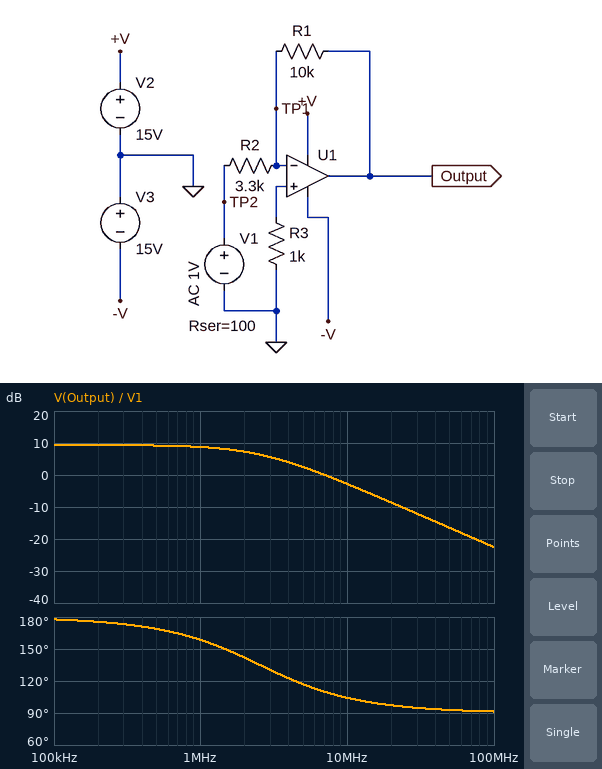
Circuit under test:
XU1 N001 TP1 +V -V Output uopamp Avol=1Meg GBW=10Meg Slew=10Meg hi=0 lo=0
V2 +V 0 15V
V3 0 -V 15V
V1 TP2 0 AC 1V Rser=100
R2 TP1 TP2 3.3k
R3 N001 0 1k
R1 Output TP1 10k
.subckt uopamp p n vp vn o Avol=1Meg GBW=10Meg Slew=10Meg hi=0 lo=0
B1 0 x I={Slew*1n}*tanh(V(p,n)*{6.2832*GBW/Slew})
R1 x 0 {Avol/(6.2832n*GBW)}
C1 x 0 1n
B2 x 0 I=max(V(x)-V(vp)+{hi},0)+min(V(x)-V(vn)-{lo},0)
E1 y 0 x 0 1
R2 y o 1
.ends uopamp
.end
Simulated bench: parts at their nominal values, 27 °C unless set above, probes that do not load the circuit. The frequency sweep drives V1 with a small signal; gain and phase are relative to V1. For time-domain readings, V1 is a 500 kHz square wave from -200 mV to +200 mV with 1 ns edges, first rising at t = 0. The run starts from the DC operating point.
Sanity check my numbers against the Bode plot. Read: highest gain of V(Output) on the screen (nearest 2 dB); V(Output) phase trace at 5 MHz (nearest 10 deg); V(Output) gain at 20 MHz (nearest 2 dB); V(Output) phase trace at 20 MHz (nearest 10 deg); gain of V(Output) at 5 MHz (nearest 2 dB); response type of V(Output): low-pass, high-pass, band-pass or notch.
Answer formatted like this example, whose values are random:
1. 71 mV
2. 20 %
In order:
1. 10 dB
2. 120 deg
3. -8 dB
4. 100 deg
5. 2 dB
6. low-pass
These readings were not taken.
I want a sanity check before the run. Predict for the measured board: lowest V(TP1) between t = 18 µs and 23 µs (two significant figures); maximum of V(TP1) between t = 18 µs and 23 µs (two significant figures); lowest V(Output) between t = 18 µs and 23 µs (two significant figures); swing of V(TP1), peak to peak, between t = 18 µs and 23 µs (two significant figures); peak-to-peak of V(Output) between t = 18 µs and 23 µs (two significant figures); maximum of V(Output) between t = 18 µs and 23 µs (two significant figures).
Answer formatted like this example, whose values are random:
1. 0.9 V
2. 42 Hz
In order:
1. -300 mV
2. 300 mV
3. -590 mV
4. 590 mV
5. 1.2 V
6. 590 mV
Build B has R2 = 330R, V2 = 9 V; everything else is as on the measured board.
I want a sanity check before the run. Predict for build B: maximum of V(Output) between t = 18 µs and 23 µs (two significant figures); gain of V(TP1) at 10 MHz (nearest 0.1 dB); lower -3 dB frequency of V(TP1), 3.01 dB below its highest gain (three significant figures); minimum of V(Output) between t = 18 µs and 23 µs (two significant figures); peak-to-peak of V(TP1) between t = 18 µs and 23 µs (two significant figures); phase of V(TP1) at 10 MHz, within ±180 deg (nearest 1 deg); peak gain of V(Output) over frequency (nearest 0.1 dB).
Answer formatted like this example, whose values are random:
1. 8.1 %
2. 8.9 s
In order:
1. 3.5 V
2. -0.4 dB
3. 412 kHz
4. -3.5 V
5. 670 mV
6. 2 deg
7. 27.3 dB
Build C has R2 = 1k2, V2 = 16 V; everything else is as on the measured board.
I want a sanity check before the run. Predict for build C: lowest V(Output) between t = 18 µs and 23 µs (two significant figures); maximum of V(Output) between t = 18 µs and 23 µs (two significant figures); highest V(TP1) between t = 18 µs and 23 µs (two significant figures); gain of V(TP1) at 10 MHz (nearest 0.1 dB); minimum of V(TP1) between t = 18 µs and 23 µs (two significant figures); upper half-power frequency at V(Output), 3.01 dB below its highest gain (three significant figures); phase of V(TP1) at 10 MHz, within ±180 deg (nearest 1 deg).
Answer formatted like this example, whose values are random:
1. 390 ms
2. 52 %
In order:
1. -1.5 V
2. 1.5 V
3. 350 mV
4. -1.1 dB
5. -350 mV
6. 1.15 MHz
7. 7 deg
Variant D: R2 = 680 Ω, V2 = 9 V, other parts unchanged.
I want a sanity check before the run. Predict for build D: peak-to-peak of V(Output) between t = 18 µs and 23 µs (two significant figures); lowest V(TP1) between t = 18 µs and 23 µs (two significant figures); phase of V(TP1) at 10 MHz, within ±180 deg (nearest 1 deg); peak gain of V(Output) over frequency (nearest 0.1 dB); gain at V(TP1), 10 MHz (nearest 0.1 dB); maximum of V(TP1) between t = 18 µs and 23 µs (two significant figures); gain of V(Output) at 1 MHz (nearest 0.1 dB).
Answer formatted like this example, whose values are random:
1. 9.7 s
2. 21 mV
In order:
1. 4.9 V
2. -360 mV
3. 4 deg
4. 22.2 dB
5. -0.7 dB
6. 360 mV
7. 17.5 dB
